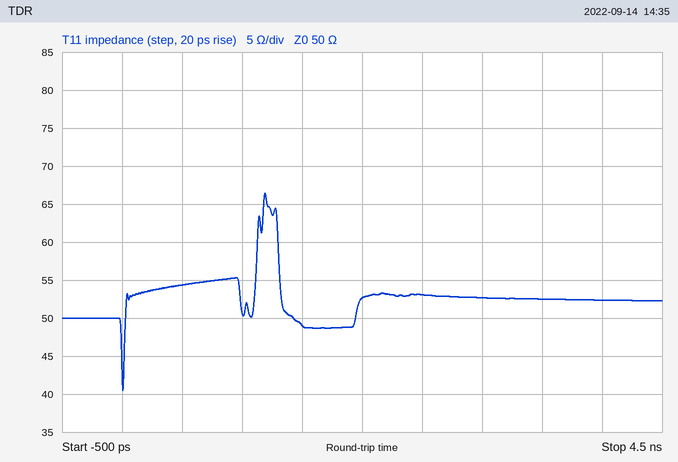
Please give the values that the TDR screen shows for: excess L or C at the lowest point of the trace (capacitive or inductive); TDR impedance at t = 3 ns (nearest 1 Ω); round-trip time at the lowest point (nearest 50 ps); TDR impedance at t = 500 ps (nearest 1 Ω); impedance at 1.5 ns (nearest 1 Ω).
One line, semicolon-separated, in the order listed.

capacitive; 53 Ω; 0 ps; 54 Ω; 49 Ω
